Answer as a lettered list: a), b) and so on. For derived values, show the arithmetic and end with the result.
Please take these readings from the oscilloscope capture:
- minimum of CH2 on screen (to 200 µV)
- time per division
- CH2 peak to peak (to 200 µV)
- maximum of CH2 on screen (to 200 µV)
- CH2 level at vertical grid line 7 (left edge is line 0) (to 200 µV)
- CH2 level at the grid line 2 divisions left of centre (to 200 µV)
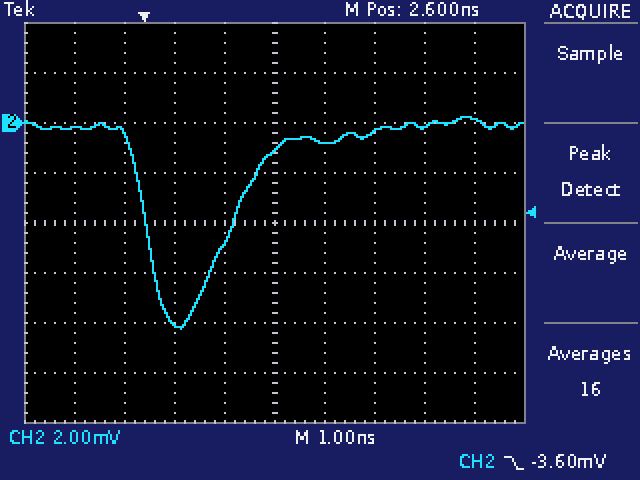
a) -8.2 mV
b) 1 ns
c) 200 µV − (-8.2 mV) = 8.4 mV
d) 200 µV
e) -400 µV
f) -8.0 mV
